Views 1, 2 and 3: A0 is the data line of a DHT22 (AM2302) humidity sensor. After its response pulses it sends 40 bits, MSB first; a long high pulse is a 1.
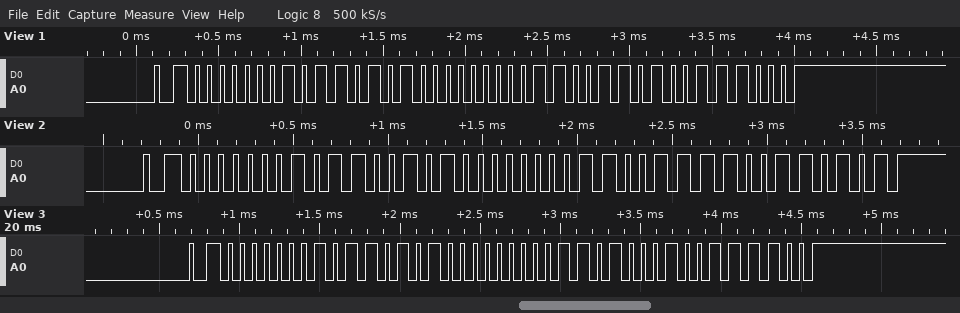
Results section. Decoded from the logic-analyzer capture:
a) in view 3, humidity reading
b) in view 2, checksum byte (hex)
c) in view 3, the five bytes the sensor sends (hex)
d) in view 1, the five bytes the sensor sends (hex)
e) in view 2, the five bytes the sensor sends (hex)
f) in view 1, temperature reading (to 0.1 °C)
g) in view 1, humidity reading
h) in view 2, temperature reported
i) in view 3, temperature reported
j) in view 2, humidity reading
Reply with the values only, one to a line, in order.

36.2 %
0x35
01 6A 00 D1 3C
01 6A 00 CD 38
01 65 00 CF 35
20.5 °C
36.2 %
20.7 °C
20.9 °C
35.7 %
